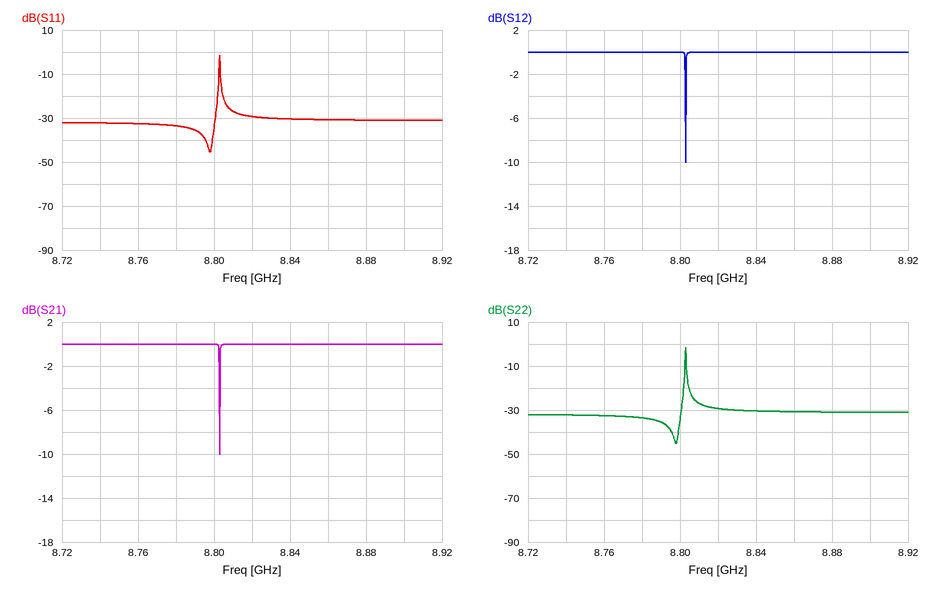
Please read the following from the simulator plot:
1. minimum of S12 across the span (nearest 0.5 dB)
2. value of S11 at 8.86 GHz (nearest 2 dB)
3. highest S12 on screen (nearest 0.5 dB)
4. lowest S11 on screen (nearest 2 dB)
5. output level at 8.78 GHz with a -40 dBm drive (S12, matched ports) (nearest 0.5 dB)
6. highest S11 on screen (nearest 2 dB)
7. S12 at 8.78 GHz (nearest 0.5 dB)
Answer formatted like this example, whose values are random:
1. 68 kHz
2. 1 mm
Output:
1. -10.0 dB
2. -30 dB
3. 0.0 dB
4. -46 dB
5. -40.0 dBm
6. -2 dB
7. 0.0 dB
